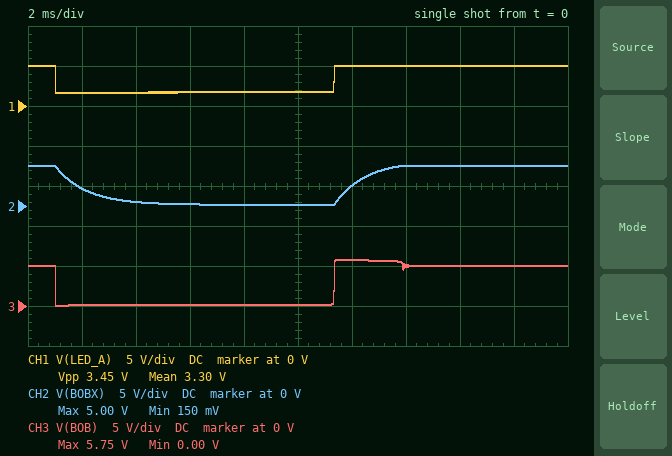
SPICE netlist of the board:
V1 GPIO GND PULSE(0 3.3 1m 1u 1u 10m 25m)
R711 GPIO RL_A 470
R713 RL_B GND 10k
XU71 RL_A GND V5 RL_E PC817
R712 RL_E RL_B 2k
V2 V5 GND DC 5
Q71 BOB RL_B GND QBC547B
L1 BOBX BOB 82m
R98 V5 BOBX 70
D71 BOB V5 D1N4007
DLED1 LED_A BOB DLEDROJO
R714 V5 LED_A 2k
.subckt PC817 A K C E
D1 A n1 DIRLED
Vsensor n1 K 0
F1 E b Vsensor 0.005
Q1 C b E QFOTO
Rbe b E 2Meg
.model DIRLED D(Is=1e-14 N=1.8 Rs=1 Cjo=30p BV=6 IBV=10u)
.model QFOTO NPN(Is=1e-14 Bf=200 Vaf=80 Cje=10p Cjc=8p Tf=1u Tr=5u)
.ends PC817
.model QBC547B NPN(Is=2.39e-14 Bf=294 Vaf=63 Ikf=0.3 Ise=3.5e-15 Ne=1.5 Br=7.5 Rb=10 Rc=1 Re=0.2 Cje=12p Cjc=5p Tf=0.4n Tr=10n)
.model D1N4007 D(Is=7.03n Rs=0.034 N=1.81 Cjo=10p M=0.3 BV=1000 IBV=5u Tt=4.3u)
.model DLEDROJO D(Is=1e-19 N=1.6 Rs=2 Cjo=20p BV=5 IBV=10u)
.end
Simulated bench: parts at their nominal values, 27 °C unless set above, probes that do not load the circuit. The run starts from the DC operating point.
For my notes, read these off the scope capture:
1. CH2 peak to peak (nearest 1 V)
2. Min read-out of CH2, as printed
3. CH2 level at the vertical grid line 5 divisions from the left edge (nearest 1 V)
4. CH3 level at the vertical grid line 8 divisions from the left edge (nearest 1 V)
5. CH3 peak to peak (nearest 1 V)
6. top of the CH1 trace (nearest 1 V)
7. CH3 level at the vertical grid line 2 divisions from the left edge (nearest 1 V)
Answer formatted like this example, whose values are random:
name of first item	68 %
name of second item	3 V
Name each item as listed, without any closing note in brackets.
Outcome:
CH2 peak to peak	5 V
Min read-out of CH2, as printed	150 mV
CH2 level at the vertical grid line 5 divisions from the left edge	0 V
CH3 level at the vertical grid line 8 divisions from the left edge	5 V
CH3 peak to peak	6 V
top of the CH1 trace	5 V
CH3 level at the vertical grid line 2 divisions from the left edge	0 V
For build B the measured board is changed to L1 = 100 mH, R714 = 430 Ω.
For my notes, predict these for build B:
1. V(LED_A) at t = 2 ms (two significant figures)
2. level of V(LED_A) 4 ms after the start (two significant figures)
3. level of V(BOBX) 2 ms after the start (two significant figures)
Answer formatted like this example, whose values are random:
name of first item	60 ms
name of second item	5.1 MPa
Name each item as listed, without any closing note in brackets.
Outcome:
V(LED_A) at t = 2 ms	1.7 V
level of V(LED_A) 4 ms after the start	1.8 V
level of V(BOBX) 2 ms after the start	2.5 V
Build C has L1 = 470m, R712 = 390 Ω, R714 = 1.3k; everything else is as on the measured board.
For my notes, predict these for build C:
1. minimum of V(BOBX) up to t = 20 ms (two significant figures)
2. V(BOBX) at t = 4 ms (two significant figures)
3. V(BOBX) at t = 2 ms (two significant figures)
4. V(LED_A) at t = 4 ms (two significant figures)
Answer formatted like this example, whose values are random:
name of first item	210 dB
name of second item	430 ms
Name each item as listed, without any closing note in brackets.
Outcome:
minimum of V(BOBX) up to t = 20 ms	1.1 V
V(BOBX) at t = 4 ms	3.2 V
V(BOBX) at t = 2 ms	4.3 V
V(LED_A) at t = 4 ms	1.6 V
